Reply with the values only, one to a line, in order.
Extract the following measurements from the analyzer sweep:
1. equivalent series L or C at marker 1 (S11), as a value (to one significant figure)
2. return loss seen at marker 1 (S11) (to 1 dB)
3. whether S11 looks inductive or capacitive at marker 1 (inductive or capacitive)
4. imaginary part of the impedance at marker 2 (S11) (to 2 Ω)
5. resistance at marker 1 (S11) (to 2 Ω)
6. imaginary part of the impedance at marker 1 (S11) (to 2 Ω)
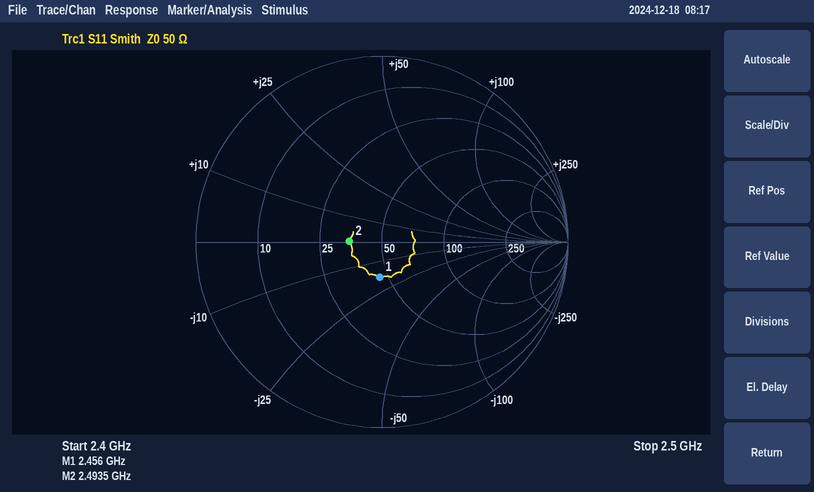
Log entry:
4 pF
14 dB
capacitive
0 Ω
46 Ω
-18 Ω
